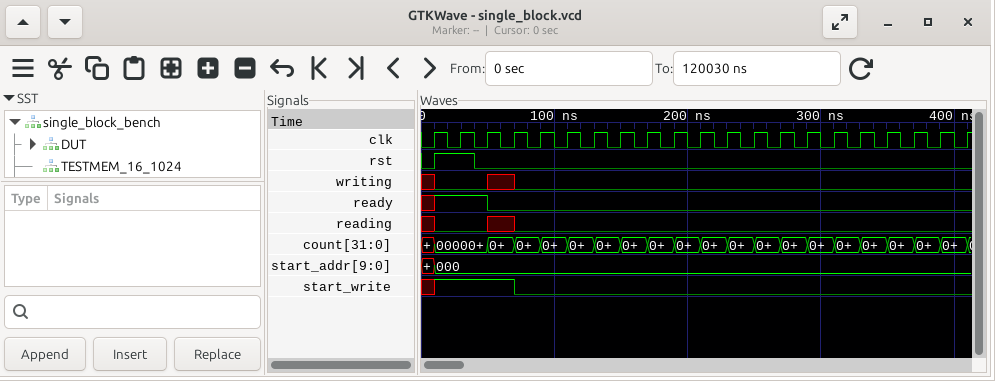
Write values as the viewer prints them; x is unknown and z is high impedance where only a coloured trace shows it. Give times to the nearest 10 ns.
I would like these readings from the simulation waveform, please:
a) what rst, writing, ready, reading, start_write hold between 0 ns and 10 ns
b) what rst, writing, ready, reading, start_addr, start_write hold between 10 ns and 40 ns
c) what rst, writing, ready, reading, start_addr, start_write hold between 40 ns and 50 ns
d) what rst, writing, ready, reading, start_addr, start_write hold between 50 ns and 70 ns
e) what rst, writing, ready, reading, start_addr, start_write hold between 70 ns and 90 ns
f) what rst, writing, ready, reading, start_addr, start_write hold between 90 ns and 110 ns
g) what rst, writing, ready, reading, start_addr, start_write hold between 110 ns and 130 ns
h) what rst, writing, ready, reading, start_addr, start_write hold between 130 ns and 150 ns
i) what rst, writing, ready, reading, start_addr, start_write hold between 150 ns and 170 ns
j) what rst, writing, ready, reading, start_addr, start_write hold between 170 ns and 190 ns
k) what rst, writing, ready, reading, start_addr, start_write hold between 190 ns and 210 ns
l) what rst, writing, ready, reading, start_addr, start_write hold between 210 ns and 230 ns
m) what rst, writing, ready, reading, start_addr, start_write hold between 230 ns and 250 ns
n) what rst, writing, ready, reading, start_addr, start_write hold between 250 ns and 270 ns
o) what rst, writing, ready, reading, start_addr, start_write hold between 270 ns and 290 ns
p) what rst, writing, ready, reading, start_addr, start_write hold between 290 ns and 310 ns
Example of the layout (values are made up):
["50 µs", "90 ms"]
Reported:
["rst=0, writing=x, ready=x, reading=x, start_write=x", "rst=1, writing=0, ready=1, reading=0, start_addr=000, start_write=1", "rst=0, writing=0, ready=1, reading=0, start_addr=000, start_write=1", "rst=0, writing=x, ready=0, reading=x, start_addr=000, start_write=1", "rst=0, writing=0, ready=0, reading=0, start_addr=000, start_write=0", "rst=0, writing=0, ready=0, reading=0, start_addr=000, start_write=0", "rst=0, writing=0, ready=0, reading=0, start_addr=000, start_write=0", "rst=0, writing=0, ready=0, reading=0, start_addr=000, start_write=0", "rst=0, writing=0, ready=0, reading=0, start_addr=000, start_write=0", "rst=0, writing=0, ready=0, reading=0, start_addr=000, start_write=0", "rst=0, writing=0, ready=0, reading=0, start_addr=000, start_write=0", "rst=0, writing=0, ready=0, reading=0, start_addr=000, start_write=0", "rst=0, writing=0, ready=0, reading=0, start_addr=000, start_write=0", "rst=0, writing=0, ready=0, reading=0, start_addr=000, start_write=0", "rst=0, writing=0, ready=0, reading=0, start_addr=000, start_write=0", "rst=0, writing=0, ready=0, reading=0, start_addr=000, start_write=0"]
